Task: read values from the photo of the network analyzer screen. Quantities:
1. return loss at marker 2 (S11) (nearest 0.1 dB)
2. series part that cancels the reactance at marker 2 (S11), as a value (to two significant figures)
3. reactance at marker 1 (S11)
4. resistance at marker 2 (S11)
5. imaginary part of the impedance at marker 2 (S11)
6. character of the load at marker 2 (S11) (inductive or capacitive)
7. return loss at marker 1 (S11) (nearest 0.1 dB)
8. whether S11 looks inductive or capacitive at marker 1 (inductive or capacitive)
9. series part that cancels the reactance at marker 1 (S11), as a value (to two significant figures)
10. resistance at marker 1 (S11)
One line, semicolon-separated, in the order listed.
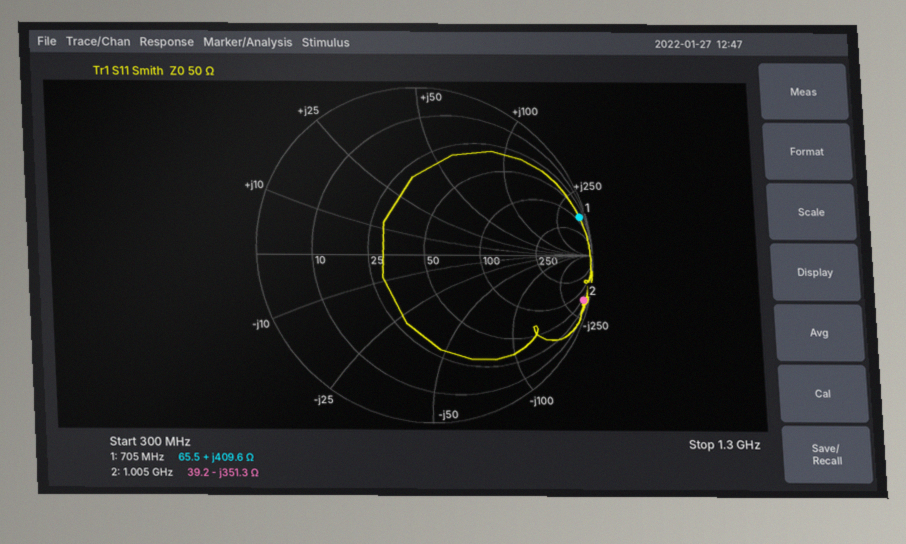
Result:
0.3 dB; 56 nH; +409.6 Ω; 39.2 Ω; -351.3 Ω; capacitive; 0.3 dB; inductive; 550 fF; 65.5 Ω
